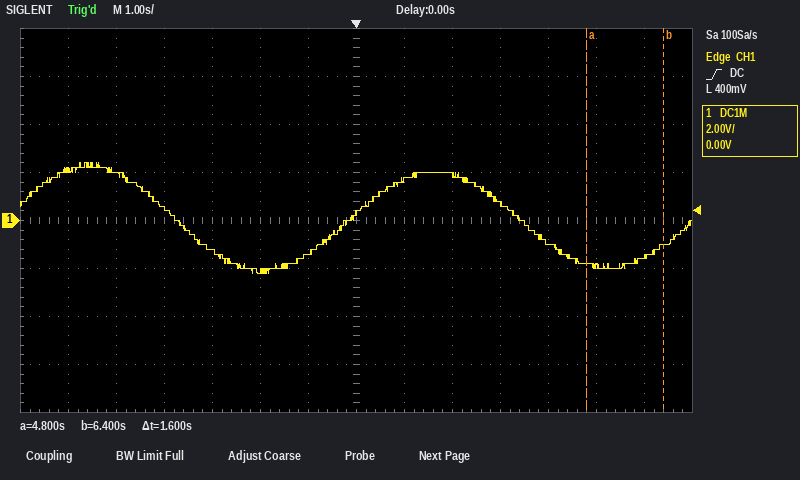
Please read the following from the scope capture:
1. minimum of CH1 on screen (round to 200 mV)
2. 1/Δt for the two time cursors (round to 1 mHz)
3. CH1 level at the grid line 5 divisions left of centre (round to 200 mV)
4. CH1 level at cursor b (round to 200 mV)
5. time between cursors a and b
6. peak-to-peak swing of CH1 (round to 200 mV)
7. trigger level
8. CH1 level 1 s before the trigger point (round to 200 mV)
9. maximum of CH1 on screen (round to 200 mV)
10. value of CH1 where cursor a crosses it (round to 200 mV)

-2.2 V
625 mHz
2.0 V
-1.0 V
1.6 s
4.6 V
400 mV
-1.4 V
2.4 V
-1.8 V
